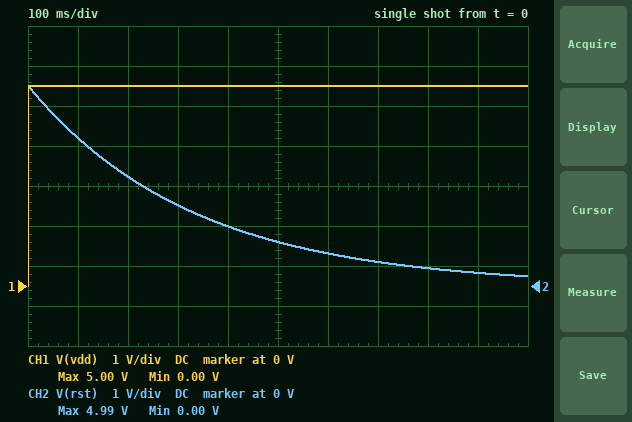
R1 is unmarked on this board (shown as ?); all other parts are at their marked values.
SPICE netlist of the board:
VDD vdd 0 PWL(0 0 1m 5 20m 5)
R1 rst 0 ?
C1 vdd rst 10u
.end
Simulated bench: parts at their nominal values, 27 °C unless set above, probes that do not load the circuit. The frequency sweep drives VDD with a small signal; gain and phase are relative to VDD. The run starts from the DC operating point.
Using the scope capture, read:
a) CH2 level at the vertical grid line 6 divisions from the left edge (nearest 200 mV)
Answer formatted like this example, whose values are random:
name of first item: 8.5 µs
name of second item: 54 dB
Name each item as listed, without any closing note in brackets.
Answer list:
CH2 level at the vertical grid line 6 divisions from the left edge: 800 mV
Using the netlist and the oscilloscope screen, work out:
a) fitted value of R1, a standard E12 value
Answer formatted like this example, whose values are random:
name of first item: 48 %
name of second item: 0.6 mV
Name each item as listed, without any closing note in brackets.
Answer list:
fitted value of R1, a standard E12 value: 33 kΩ
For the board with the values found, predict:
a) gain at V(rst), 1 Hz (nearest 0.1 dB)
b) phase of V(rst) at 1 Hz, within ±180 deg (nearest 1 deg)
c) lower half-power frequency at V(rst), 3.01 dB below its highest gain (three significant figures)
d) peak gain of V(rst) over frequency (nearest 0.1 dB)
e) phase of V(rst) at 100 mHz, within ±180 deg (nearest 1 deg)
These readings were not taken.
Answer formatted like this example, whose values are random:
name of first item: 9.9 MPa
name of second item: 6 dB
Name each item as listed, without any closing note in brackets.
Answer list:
gain at V(rst), 1 Hz: -0.9 dB
phase of V(rst) at 1 Hz, within ±180 deg: 26 deg
lower half-power frequency at V(rst), 3.01 dB below its highest gain: 482 mHz
peak gain of V(rst) over frequency: 0 dB
phase of V(rst) at 100 mHz, within ±180 deg: 78 deg
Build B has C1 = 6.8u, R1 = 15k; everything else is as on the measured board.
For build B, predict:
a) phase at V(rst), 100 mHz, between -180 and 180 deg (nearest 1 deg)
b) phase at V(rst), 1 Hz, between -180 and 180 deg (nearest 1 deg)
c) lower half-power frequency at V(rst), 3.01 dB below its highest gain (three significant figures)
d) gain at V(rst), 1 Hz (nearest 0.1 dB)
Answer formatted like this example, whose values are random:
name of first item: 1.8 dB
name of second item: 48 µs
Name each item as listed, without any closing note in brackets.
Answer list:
phase at V(rst), 100 mHz, between -180 and 180 deg: 86 deg
phase at V(rst), 1 Hz, between -180 and 180 deg: 57 deg
lower half-power frequency at V(rst), 3.01 dB below its highest gain: 1.56 Hz
gain at V(rst), 1 Hz: -5.4 dB
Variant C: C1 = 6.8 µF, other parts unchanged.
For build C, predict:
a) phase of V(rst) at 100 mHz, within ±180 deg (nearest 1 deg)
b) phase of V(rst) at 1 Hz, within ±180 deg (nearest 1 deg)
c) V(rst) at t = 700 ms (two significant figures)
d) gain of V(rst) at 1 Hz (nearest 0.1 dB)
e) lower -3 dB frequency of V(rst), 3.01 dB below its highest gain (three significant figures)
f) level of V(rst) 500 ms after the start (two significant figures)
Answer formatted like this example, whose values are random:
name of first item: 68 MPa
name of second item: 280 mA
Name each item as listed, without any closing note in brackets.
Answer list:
phase of V(rst) at 100 mHz, within ±180 deg: 82 deg
phase of V(rst) at 1 Hz, within ±180 deg: 35 deg
V(rst) at t = 700 ms: 220 mV
gain of V(rst) at 1 Hz: -1.8 dB
lower -3 dB frequency of V(rst), 3.01 dB below its highest gain: 709 mHz
level of V(rst) 500 ms after the start: 540 mV
